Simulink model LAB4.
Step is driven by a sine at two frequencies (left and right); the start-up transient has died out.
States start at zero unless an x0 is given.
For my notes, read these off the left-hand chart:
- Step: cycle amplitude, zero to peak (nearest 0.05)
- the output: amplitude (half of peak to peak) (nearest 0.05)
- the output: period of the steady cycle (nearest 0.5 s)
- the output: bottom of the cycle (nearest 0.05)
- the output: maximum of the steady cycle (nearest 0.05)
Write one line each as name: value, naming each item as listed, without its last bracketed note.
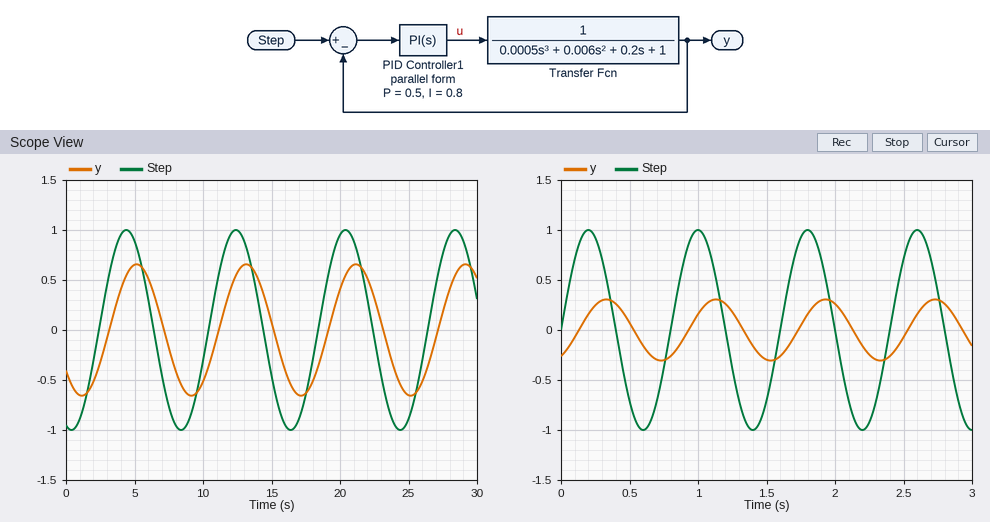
Step: cycle amplitude, zero to peak: 1.00
the output: amplitude (half of peak to peak): 0.65
the output: period of the steady cycle: 8.0 s
the output: bottom of the cycle: -0.65
the output: maximum of the steady cycle: 0.65
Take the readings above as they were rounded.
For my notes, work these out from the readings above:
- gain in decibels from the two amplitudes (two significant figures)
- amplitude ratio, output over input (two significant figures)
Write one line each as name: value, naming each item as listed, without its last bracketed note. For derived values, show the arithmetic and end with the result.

gain in decibels from the two amplitudes: 20 log10(0.65 / 1) = -3.7 dB
amplitude ratio, output over input: 0.65 / 1 = 0.65
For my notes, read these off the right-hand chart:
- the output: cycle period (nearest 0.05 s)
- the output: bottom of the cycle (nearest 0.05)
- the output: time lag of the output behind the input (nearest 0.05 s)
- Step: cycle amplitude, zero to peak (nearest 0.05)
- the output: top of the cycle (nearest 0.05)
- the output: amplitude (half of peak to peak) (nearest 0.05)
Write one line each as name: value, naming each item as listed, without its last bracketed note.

the output: cycle period: 0.80 s
the output: bottom of the cycle: -0.30
the output: time lag of the output behind the input: 0.15 s
Step: cycle amplitude, zero to peak: 1.00
the output: top of the cycle: 0.30
the output: amplitude (half of peak to peak): 0.30
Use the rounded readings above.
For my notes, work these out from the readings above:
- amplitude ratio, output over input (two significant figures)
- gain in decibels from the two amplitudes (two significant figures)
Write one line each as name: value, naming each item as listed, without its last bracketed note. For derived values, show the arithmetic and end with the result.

amplitude ratio, output over input: 0.3 / 1 = 0.30
gain in decibels from the two amplitudes: 20 log10(0.3 / 1) = -10 dB
